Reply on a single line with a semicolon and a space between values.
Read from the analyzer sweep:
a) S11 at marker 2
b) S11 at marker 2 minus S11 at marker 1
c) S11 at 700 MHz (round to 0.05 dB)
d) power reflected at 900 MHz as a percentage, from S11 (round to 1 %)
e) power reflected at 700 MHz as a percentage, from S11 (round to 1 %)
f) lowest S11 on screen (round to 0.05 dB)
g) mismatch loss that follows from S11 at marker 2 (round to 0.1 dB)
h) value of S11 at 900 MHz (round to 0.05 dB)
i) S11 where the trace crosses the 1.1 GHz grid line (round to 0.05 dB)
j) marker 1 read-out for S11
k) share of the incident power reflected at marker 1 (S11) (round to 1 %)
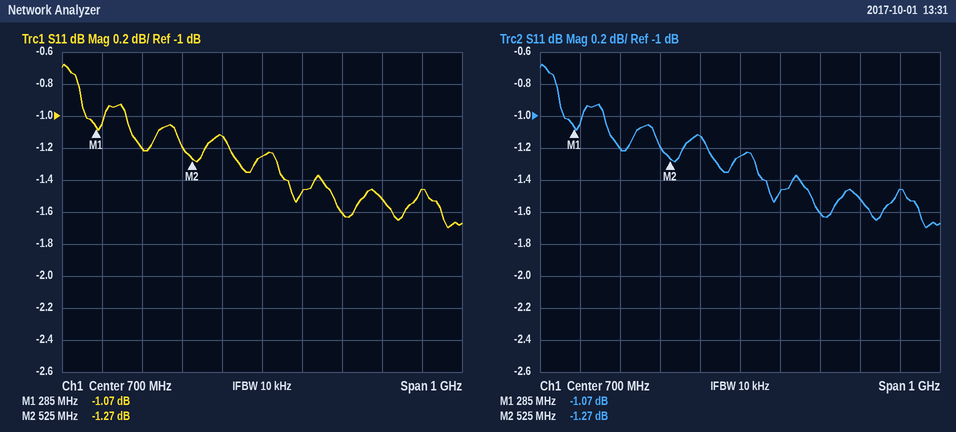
-1.27 dB; -0.20 dB; -1.25 dB; 69 %; 75 %; -1.70 dB; 6.0 dB; -1.60 dB; -1.45 dB; -1.07 dB; 78 %
